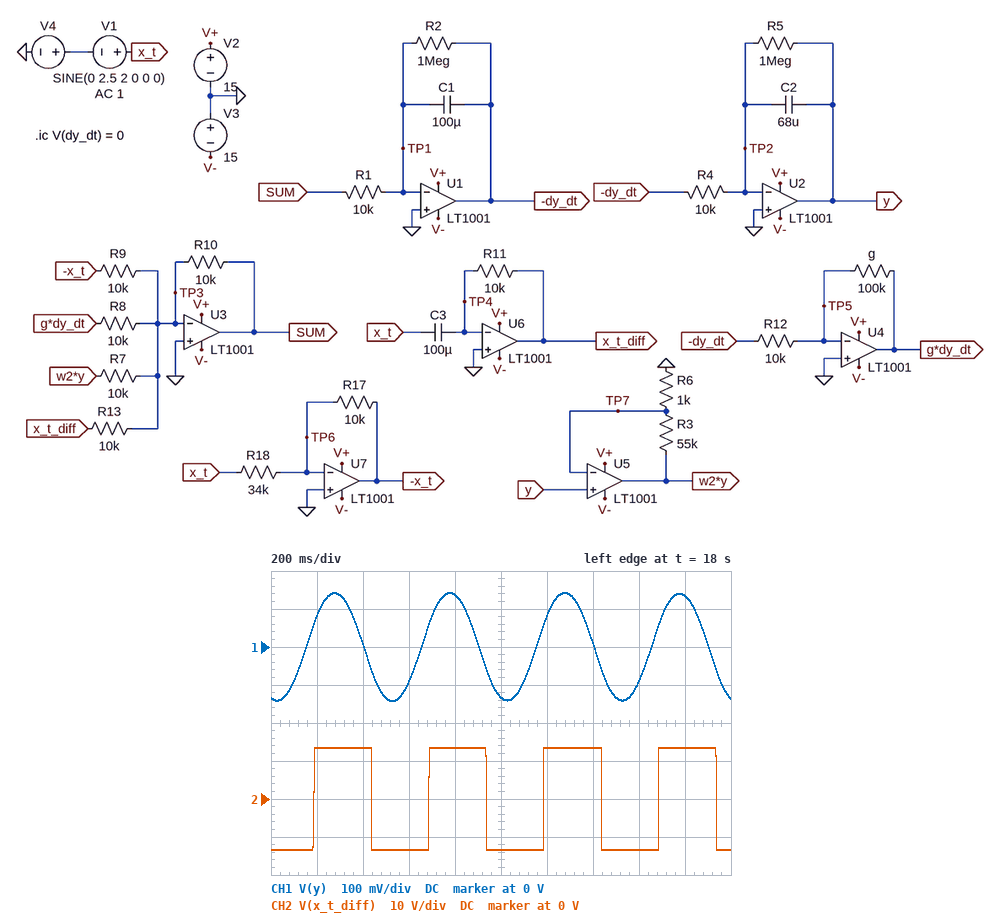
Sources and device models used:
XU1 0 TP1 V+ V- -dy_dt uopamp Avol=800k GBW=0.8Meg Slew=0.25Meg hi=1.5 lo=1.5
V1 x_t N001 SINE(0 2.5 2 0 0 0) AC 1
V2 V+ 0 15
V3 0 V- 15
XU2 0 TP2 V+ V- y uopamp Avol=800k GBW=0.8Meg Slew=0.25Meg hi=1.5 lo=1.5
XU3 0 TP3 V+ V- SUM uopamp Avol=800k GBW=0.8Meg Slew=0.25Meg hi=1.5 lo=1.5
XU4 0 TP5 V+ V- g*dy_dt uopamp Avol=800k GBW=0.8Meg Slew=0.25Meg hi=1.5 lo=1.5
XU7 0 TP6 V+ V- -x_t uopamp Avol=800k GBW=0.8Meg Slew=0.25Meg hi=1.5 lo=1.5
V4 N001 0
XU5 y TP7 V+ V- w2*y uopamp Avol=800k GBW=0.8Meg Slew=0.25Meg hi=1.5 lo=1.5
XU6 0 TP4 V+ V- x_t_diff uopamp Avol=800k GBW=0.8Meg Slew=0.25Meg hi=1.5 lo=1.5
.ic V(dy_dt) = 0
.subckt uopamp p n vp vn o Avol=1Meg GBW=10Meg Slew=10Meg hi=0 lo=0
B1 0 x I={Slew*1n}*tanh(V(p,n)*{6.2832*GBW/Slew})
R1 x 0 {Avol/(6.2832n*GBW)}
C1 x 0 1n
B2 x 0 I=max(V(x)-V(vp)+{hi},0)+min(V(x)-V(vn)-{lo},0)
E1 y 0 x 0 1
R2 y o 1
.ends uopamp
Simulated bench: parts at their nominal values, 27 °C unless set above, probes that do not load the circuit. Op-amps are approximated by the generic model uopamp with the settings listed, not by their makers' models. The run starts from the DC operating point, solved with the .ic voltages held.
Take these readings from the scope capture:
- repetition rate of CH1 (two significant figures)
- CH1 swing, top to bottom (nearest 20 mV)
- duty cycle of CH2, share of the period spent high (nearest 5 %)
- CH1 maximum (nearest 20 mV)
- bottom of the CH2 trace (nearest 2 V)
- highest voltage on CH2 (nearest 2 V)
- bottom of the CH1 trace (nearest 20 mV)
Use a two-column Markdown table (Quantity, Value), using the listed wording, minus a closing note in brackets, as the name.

| Quantity | Value |
|---|---|
| repetition rate of CH1 | 2.0 Hz |
| CH1 swing, top to bottom | 280 mV |
| duty cycle of CH2, share of the period spent high | 50 % |
| CH1 maximum | 140 mV |
| bottom of the CH2 trace | -14 V |
| highest voltage on CH2 | 14 V |
| bottom of the CH1 trace | -140 mV |
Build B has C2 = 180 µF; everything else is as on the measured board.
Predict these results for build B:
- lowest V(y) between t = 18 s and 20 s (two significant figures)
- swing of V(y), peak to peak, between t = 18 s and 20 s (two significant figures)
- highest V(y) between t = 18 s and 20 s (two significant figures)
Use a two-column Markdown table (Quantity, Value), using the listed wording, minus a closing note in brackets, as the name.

| Quantity | Value |
|---|---|
| lowest V(y) between t = 18 s and 20 s | -50 mV |
| swing of V(y), peak to peak, between t = 18 s and 20 s | 100 mV |
| highest V(y) between t = 18 s and 20 s | 50 mV |
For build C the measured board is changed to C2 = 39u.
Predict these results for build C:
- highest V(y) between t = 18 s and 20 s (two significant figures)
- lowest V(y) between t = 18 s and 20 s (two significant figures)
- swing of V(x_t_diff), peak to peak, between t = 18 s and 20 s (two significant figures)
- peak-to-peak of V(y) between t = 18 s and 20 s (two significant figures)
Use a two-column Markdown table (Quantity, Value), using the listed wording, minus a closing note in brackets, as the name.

| Quantity | Value |
|---|---|
| highest V(y) between t = 18 s and 20 s | 260 mV |
| lowest V(y) between t = 18 s and 20 s | -260 mV |
| swing of V(x_t_diff), peak to peak, between t = 18 s and 20 s | 27 V |
| peak-to-peak of V(y) between t = 18 s and 20 s | 510 mV |
